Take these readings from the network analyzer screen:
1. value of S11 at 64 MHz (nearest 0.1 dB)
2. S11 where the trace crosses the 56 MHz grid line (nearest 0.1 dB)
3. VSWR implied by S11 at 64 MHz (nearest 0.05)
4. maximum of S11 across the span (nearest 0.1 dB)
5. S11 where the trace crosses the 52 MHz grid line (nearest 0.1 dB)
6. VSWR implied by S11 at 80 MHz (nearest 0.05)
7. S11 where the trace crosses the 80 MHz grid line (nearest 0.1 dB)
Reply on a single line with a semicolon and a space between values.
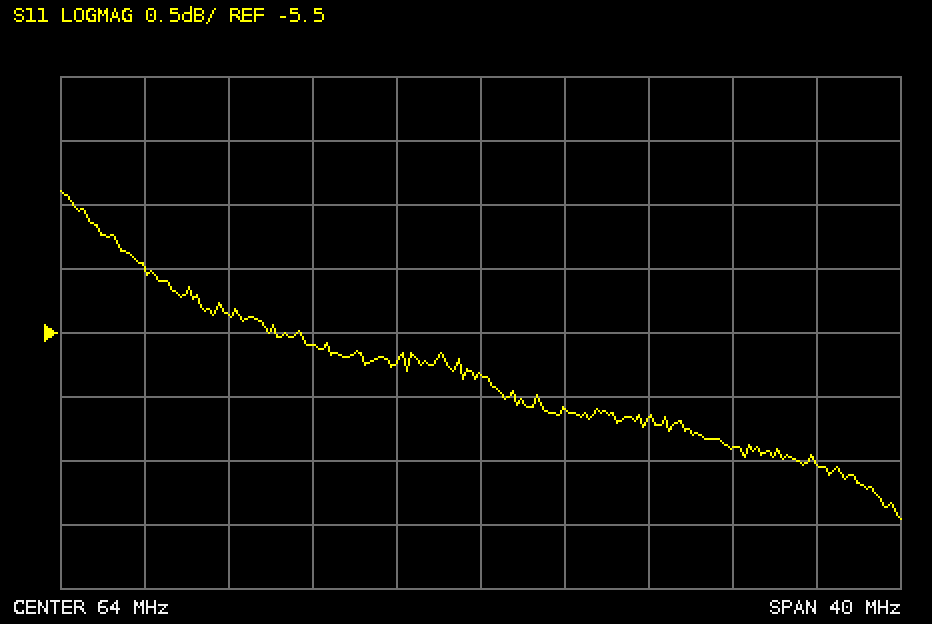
-5.8 dB; -5.6 dB; 3.10; -4.4 dB; -5.4 dB; 2.80; -6.5 dB
